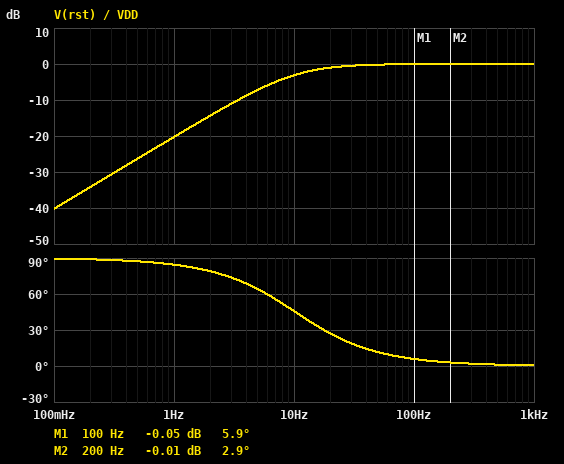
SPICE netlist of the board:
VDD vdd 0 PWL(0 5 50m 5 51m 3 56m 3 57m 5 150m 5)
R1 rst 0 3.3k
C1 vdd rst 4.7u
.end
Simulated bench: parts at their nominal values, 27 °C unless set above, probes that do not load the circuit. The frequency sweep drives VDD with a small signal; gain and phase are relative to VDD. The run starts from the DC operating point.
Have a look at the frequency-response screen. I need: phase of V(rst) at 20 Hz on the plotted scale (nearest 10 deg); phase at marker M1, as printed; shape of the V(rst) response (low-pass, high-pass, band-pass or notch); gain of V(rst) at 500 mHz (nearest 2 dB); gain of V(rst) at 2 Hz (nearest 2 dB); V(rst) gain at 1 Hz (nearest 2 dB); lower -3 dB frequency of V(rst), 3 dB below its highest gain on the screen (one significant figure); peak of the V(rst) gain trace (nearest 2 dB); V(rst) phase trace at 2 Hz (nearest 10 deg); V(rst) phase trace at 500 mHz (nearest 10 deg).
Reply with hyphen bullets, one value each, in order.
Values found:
- 30 deg
- 5.9 deg
- high-pass
- -26 dB
- -14 dB
- -20 dB
- 10 Hz
- 0 dB
- 80 deg
- 90 deg
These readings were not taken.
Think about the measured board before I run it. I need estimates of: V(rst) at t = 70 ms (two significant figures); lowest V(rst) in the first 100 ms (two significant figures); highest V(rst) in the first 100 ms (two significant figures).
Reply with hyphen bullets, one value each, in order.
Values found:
- 270 mV
- -1.9 V
- 620 mV
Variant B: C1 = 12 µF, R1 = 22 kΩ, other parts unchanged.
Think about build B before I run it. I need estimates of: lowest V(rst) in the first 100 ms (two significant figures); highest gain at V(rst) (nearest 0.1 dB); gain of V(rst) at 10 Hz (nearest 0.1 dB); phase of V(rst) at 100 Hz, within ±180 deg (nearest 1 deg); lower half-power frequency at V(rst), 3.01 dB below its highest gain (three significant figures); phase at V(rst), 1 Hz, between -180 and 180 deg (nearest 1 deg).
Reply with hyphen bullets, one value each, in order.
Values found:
- -2.0 V
- 0 dB
- 0 dB
- 0 deg
- 603 mHz
- 31 deg
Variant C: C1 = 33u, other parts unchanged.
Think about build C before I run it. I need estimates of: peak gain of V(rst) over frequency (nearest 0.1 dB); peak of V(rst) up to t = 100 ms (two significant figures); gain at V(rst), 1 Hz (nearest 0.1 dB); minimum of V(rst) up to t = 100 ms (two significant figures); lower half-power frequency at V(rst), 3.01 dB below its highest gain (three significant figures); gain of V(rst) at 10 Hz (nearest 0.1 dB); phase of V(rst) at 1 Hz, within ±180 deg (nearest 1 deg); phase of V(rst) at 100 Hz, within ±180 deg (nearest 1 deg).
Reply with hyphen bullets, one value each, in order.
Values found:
- 0 dB
- 110 mV
- -5.0 dB
- -2.0 V
- 1.46 Hz
- -0.1 dB
- 56 deg
- 1 deg
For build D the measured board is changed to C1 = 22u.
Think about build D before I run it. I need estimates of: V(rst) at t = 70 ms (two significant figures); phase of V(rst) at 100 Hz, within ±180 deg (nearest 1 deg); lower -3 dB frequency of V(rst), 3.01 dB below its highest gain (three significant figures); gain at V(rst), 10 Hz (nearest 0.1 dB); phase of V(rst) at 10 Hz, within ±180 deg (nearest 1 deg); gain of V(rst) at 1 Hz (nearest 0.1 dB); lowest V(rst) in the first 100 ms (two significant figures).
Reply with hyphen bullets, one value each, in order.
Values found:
- 130 mV
- 1 deg
- 2.19 Hz
- -0.2 dB
- 12 deg
- -7.6 dB
- -2.0 V
